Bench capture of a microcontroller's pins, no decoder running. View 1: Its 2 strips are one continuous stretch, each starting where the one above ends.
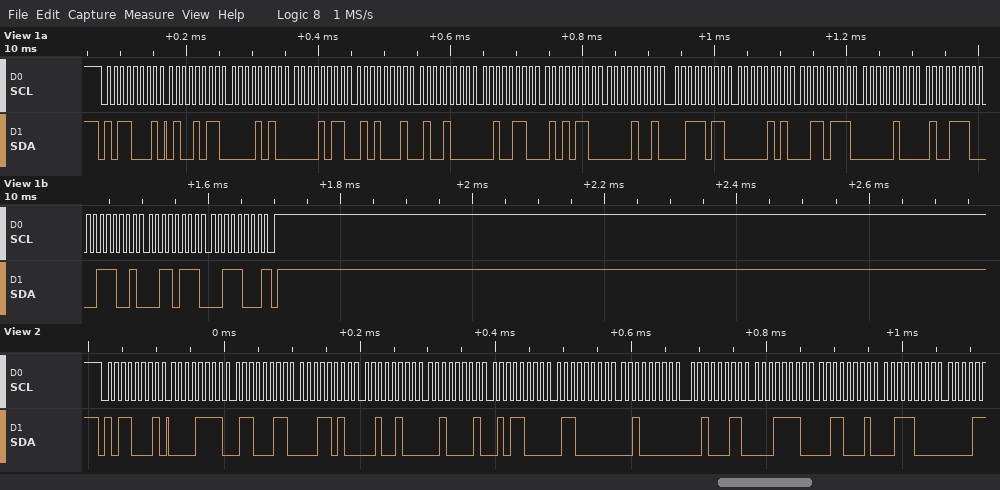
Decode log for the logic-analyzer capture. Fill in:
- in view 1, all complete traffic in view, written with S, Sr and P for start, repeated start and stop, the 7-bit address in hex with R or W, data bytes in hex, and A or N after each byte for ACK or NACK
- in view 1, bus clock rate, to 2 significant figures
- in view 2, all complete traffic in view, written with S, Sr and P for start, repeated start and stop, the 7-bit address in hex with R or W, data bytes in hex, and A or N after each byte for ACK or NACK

S 58R A 4B A 0A A 0B A 51 A 48 A 26 A 56 A 09 A 3B A 05 A 37 A 04 A 4E A 39 A 37 A 38 N P
100 kHz
S 58R A 0F A 63 A 1A A 24 A 21 A 58 A 60 A 20 A 23 A 1E A 31 A 38 A
